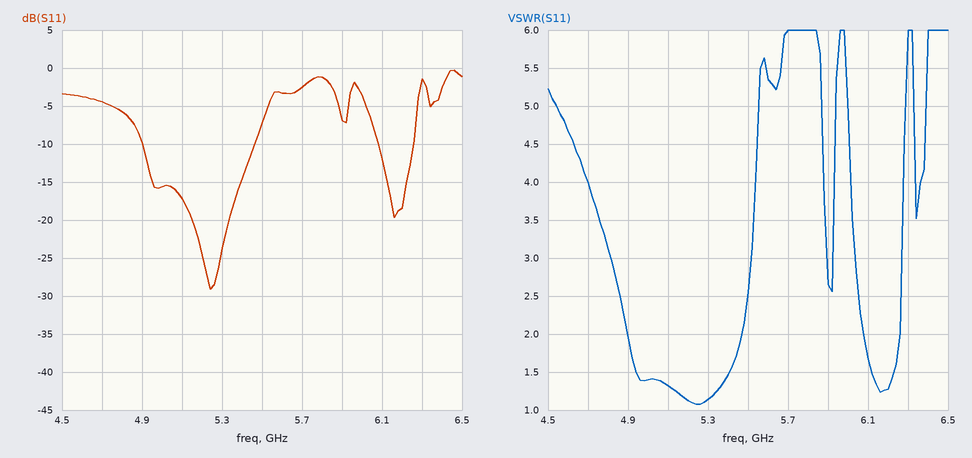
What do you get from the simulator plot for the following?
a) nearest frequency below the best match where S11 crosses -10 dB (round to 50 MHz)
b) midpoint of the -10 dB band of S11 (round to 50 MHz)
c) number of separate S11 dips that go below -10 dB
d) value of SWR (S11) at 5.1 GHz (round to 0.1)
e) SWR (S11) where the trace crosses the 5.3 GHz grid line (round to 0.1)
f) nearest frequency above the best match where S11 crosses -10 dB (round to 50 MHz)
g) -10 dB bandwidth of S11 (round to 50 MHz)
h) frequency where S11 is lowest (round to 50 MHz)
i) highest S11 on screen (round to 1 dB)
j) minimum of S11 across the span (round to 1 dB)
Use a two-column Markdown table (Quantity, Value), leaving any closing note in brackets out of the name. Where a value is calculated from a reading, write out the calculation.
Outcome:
| Quantity | Value |
|---|---|
| nearest frequency below the best match where S11 crosses -10 dB | 4.90 GHz |
| midpoint of the -10 dB band of S11 | 5.20 GHz |
| number of separate S11 dips that go below -10 dB | 2 |
| value of SWR (S11) at 5.1 GHz | 1.3 |
| SWR (S11) where the trace crosses the 5.3 GHz grid line | 1.1 |
| nearest frequency above the best match where S11 crosses -10 dB | 5.45 GHz |
| -10 dB bandwidth of S11 | 5.45 GHz − 4.90 GHz = 550 MHz |
| frequency where S11 is lowest | 5.25 GHz |
| highest S11 on screen | 0 dB |
| minimum of S11 across the span | -29 dB |
